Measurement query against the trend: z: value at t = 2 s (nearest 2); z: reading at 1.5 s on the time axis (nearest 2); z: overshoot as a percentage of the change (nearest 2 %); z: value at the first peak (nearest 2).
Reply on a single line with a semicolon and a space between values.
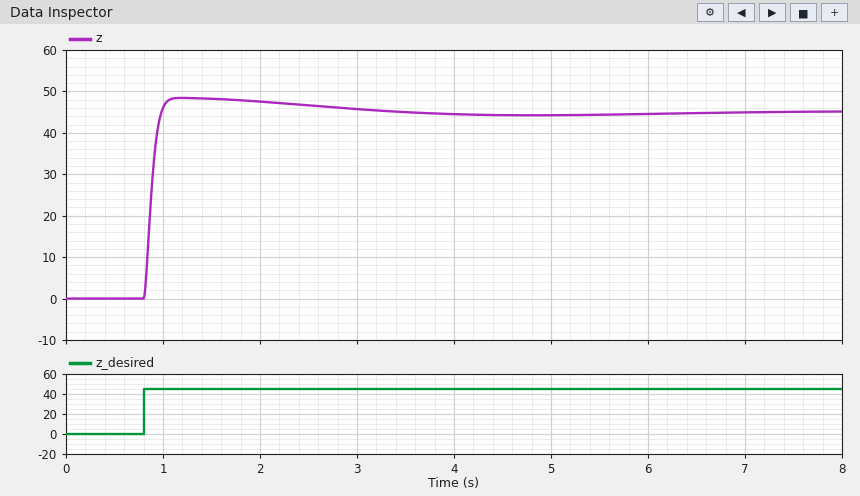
48; 48; 8 %; 48
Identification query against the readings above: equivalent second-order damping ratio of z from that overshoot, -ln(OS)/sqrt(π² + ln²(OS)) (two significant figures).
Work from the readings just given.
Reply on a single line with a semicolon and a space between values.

0.63
